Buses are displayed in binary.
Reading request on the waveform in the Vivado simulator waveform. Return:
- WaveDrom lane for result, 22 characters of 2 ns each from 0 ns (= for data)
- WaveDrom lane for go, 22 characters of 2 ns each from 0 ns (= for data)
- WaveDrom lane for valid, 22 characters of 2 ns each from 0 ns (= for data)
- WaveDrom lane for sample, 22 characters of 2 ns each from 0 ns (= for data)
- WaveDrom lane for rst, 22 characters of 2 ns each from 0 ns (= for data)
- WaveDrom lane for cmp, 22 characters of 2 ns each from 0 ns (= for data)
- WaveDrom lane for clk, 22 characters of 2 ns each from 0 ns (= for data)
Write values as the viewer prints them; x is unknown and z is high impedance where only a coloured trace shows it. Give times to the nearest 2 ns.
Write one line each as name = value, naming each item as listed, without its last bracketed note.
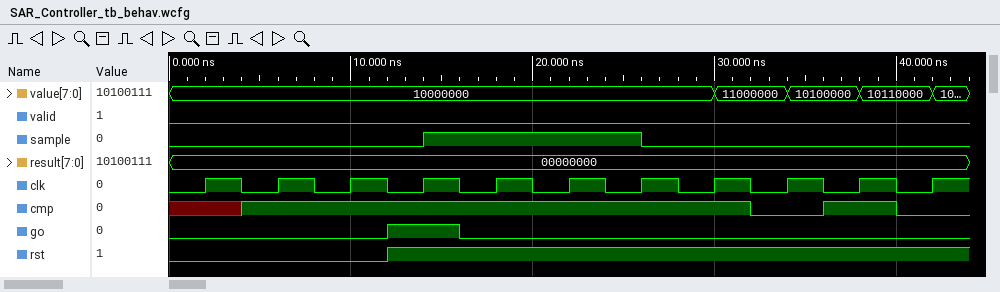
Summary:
WaveDrom lane for result, 22 characters of 2 ns each from 0 ns = {name: 'result', wave: '=.....................', data: '00000000'}
WaveDrom lane for go, 22 characters of 2 ns each from 0 ns = {name: 'go', wave: '0.....1.0.............'}
WaveDrom lane for valid, 22 characters of 2 ns each from 0 ns = {name: 'valid', wave: '0.....................'}
WaveDrom lane for sample, 22 characters of 2 ns each from 0 ns = {name: 'sample', wave: '0......1.....0........'}
WaveDrom lane for rst, 22 characters of 2 ns each from 0 ns = {name: 'rst', wave: '0.....1...............'}
WaveDrom lane for cmp, 22 characters of 2 ns each from 0 ns = {name: 'cmp', wave: 'x.1.............0.1.0.'}
WaveDrom lane for clk, 22 characters of 2 ns each from 0 ns = {name: 'clk', wave: '0101010101010101010101'}
